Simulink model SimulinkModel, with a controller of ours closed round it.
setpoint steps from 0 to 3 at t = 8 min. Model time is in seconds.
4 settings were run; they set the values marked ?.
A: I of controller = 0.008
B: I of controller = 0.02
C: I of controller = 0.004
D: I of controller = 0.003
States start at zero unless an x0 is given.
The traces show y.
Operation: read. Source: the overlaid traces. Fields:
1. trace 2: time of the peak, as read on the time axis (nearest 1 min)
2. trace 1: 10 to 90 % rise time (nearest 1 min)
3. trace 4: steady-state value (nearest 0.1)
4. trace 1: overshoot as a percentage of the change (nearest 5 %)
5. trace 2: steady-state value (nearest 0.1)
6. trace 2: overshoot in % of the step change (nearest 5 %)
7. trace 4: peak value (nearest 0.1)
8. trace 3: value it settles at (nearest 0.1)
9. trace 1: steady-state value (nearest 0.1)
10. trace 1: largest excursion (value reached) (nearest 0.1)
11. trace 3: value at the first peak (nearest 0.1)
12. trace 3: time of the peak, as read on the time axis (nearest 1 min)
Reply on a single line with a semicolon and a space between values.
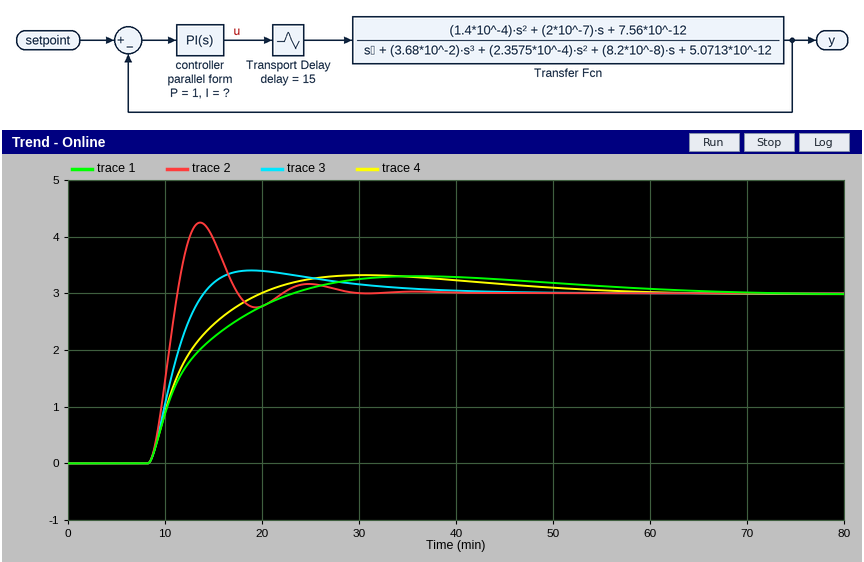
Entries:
14 min; 10 min; 3.0; 10 %; 3.0; 40 %; 3.3; 3.0; 3.0; 3.3; 3.4; 19 min
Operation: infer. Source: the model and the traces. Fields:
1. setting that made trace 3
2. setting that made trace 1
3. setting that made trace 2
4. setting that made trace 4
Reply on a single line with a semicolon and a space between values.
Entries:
A; D; B; C
